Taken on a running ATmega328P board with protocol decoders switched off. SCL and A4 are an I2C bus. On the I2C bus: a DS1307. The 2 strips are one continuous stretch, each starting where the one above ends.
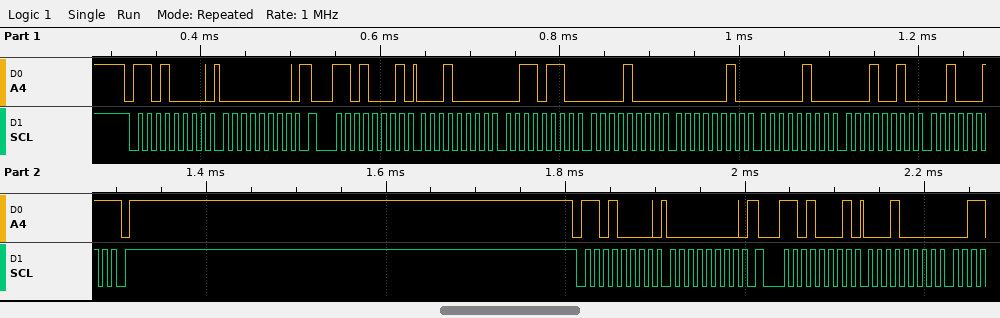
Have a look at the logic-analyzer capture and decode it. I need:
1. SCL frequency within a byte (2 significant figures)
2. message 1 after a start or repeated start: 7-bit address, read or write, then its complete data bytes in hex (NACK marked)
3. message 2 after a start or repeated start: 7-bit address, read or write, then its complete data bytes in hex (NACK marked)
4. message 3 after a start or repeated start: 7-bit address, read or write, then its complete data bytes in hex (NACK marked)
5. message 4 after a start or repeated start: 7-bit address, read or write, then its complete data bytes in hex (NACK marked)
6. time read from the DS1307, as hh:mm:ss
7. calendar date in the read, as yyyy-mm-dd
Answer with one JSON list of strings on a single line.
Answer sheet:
["100 kHz", "0x68 write: 00", "0x68 read: 10 36 08 02 04 12 23 NACK", "0x68 write: 00", "0x68 read: 10", "08:36:10", "2023-12-04"]
